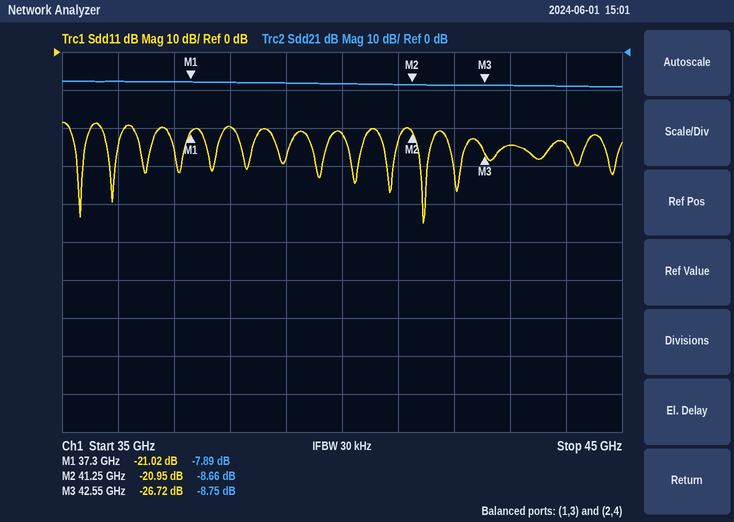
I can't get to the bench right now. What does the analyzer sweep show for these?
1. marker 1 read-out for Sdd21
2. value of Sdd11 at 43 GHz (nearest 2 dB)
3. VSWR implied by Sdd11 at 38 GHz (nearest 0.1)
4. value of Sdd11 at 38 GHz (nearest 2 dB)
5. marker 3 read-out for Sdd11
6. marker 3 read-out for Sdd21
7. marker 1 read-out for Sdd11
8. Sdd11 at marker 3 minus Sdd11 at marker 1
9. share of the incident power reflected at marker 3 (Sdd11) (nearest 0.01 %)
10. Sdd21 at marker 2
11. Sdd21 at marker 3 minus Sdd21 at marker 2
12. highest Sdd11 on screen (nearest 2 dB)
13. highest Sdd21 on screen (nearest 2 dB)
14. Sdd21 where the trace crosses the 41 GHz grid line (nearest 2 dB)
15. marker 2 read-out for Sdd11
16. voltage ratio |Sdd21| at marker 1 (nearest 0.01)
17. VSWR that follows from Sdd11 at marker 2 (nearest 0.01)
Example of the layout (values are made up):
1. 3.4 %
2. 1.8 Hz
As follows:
1. -7.89 dB
2. -24 dB
3. 1.2
4. -20 dB
5. -26.72 dB
6. -8.75 dB
7. -21.02 dB
8. -5.70 dB
9. 0.21 %
10. -8.66 dB
11. -0.09 dB
12. -18 dB
13. -8 dB
14. -8 dB
15. -20.95 dB
16. 0.40
17. 1.20
